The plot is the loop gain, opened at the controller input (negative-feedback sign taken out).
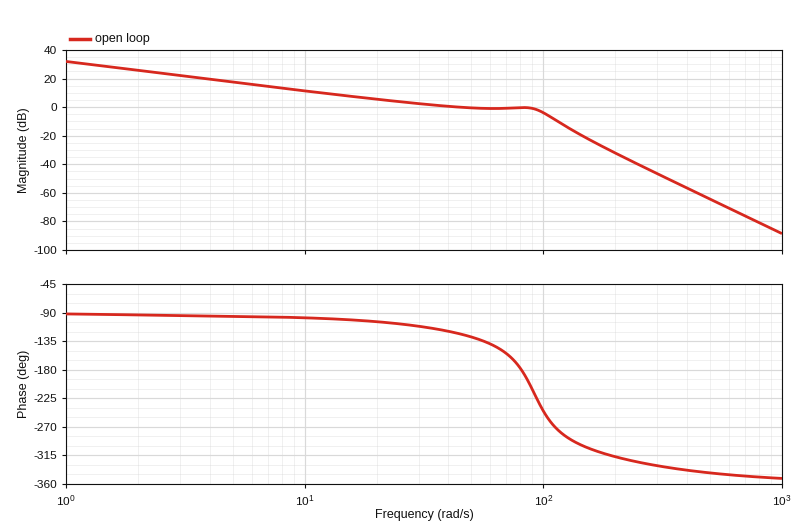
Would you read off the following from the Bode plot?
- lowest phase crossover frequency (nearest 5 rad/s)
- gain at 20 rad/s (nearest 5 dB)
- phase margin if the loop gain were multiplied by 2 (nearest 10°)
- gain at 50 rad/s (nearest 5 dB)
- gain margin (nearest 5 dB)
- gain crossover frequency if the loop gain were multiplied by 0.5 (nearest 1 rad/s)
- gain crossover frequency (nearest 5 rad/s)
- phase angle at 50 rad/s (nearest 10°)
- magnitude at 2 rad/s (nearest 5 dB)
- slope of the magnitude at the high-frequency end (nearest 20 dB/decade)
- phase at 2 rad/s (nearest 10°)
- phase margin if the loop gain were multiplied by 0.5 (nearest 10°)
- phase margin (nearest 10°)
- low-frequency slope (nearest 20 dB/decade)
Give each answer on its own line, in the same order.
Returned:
80 rad/s
5 dB
-80°
0 dB
0 dB
19 rad/s
45 rad/s
-130°
25 dB
-80 dB/decade
-90°
80°
60°
-20 dB/decade
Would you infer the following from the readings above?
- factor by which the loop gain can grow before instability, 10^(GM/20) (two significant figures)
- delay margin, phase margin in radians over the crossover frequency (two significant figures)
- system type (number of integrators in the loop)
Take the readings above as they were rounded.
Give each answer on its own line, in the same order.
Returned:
1.0
0.023 s
1
